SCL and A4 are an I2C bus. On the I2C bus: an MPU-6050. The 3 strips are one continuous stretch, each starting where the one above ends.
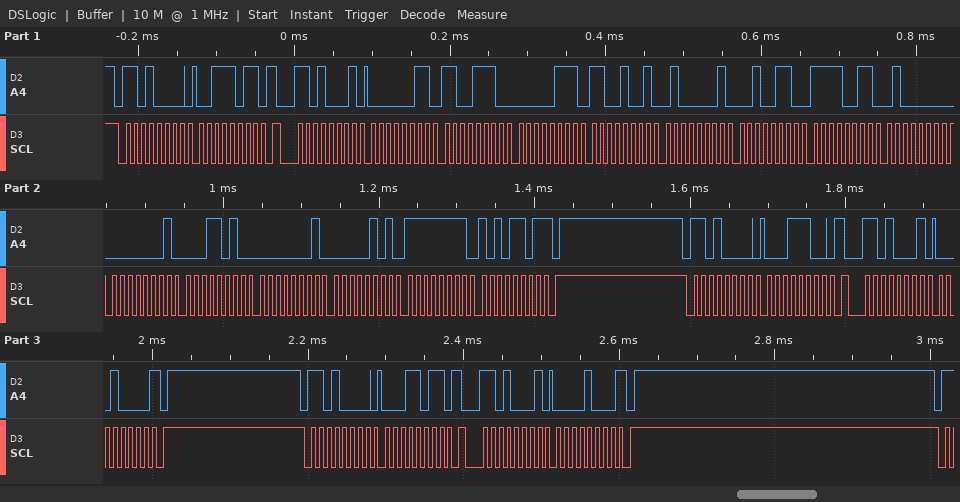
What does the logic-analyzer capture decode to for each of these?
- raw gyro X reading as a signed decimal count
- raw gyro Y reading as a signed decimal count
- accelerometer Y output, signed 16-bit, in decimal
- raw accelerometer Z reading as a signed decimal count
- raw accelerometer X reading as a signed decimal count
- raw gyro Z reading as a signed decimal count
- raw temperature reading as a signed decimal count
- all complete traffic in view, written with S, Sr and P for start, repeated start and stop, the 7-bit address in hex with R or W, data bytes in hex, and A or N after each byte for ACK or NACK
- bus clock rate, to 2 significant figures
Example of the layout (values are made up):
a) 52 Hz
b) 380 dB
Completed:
a) 282
b) 261
c) 1993
d) 16678
e) 974
f) -83
g) -3264
h) S 68W A 3B A Sr 68R A 03 A CE A 07 A C9 A 41 A 26 A F3 A 40 A 01 A 1A A 01 A 05 A FF A AD N P S 68W A 1C A Sr 68R A 10 N P S 68W A 1B A Sr 68R A 08 N P
i) 100 kHz
